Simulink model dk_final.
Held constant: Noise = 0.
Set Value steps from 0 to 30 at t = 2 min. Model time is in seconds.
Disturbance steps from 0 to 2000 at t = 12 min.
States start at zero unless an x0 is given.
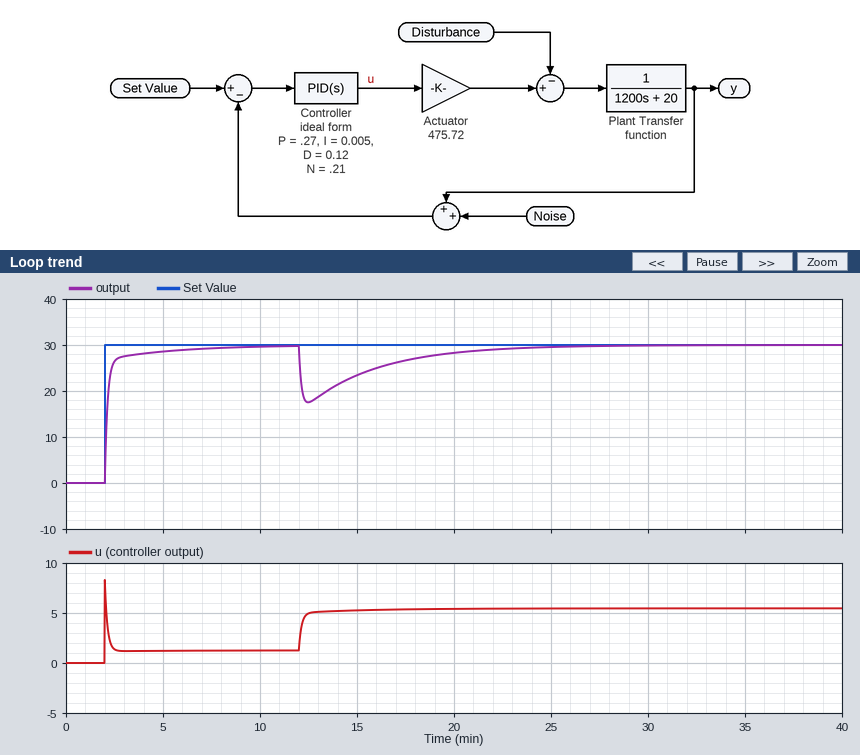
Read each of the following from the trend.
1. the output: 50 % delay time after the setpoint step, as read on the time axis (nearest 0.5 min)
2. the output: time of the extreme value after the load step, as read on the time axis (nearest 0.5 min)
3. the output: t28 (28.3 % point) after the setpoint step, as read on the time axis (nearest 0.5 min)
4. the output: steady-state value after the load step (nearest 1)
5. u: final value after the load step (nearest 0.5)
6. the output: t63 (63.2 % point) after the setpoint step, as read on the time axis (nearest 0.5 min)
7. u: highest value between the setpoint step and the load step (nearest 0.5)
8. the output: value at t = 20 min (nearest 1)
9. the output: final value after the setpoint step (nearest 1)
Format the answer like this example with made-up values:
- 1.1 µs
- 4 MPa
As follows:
- 2.0 min
- 12.5 min
- 2.0 min
- 30
- 5.5
- 2.0 min
- 8.5
- 28
- 30
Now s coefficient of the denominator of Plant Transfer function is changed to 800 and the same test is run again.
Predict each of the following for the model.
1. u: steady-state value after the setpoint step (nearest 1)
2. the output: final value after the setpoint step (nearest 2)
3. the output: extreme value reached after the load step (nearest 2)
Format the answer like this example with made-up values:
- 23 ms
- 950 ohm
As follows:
- 1
- 30
- 18
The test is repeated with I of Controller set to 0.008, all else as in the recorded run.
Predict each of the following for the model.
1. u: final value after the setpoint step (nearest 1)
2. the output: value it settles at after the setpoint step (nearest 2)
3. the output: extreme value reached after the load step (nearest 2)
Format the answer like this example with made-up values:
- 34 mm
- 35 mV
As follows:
- 1
- 30
- 18
